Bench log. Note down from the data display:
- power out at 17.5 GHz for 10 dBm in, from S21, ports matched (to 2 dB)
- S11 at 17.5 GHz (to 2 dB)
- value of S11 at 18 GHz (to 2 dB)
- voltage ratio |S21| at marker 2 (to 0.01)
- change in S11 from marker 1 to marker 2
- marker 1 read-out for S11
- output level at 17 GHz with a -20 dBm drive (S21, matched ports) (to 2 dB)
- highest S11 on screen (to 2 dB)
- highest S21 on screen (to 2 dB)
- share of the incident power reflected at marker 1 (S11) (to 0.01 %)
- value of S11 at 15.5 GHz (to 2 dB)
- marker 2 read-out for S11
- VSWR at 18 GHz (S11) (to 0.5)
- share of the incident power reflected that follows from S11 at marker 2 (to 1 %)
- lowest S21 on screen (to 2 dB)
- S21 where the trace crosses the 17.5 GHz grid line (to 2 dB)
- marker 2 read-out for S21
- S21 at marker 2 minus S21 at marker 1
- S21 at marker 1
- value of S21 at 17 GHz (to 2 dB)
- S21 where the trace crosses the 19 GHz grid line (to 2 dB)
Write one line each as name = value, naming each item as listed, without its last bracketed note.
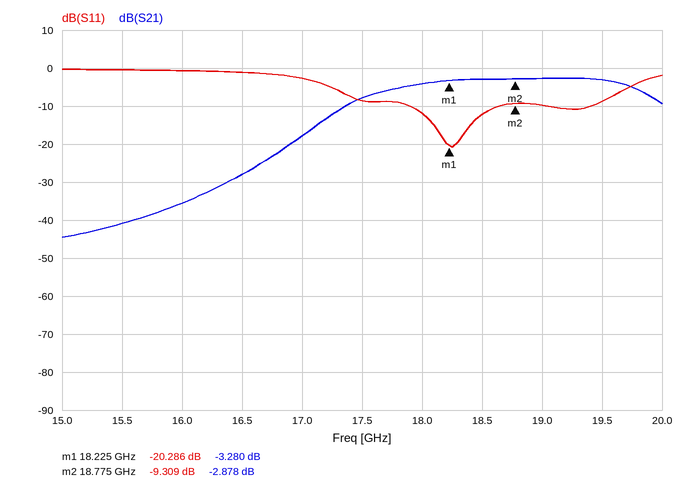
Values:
power out at 17.5 GHz for 10 dBm in, from S21, ports matched = 2 dBm
S11 at 17.5 GHz = -8 dB
value of S11 at 18 GHz = -12 dB
voltage ratio |S21| at marker 2 = 0.72
change in S11 from marker 1 to marker 2 = 10.977 dB
marker 1 read-out for S11 = -20.286 dB
output level at 17 GHz with a -20 dBm drive (S21, matched ports) = -38 dBm
highest S11 on screen = 0 dB
highest S21 on screen = -2 dB
share of the incident power reflected at marker 1 (S11) = 0.94 %
value of S11 at 15.5 GHz = 0 dB
marker 2 read-out for S11 = -9.309 dB
VSWR at 18 GHz (S11) = 1.5
share of the incident power reflected that follows from S11 at marker 2 = 12 %
lowest S21 on screen = -44 dB
S21 where the trace crosses the 17.5 GHz grid line = -8 dB
marker 2 read-out for S21 = -2.878 dB
S21 at marker 2 minus S21 at marker 1 = 0.402 dB
S21 at marker 1 = -3.280 dB
value of S21 at 17 GHz = -18 dB
S21 where the trace crosses the 19 GHz grid line = -2 dB
